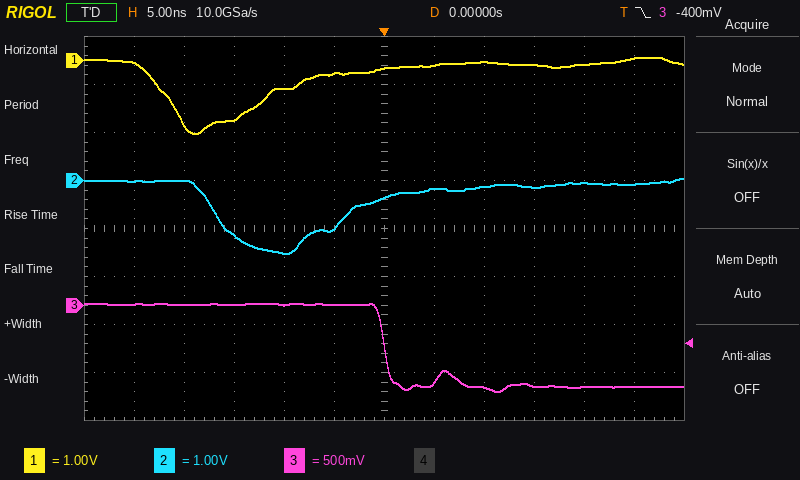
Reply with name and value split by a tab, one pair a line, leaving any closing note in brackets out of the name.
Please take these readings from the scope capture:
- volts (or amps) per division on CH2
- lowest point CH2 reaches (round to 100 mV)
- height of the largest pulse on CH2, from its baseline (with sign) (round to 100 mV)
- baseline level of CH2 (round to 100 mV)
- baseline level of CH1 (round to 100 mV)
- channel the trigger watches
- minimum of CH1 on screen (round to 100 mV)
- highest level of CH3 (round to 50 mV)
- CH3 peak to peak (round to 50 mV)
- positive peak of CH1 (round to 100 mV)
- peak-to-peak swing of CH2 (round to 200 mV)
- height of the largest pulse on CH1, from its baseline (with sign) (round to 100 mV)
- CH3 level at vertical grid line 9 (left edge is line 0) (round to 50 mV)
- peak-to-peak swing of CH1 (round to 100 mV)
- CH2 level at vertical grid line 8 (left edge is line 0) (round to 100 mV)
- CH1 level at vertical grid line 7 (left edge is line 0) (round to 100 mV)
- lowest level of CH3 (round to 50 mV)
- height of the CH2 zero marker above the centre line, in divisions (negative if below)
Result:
volts (or amps) per division on CH2	1 V
lowest point CH2 reaches	-1.5 V
height of the largest pulse on CH2, from its baseline (with sign)	-1.4 V
baseline level of CH2	-100 mV
baseline level of CH1	-100 mV
channel the trigger watches	CH3
minimum of CH1 on screen	-1.5 V
highest level of CH3	0 mV
CH3 peak to peak	900 mV
positive peak of CH1	100 mV
peak-to-peak swing of CH2	1.6 V
height of the largest pulse on CH1, from its baseline (with sign)	-1.4 V
CH3 level at vertical grid line 9 (left edge is line 0)	-850 mV
peak-to-peak swing of CH1	1.6 V
CH2 level at vertical grid line 8 (left edge is line 0)	-100 mV
CH1 level at vertical grid line 7 (left edge is line 0)	-100 mV
lowest level of CH3	-900 mV
height of the CH2 zero marker above the centre line, in divisions	+1.0 div
